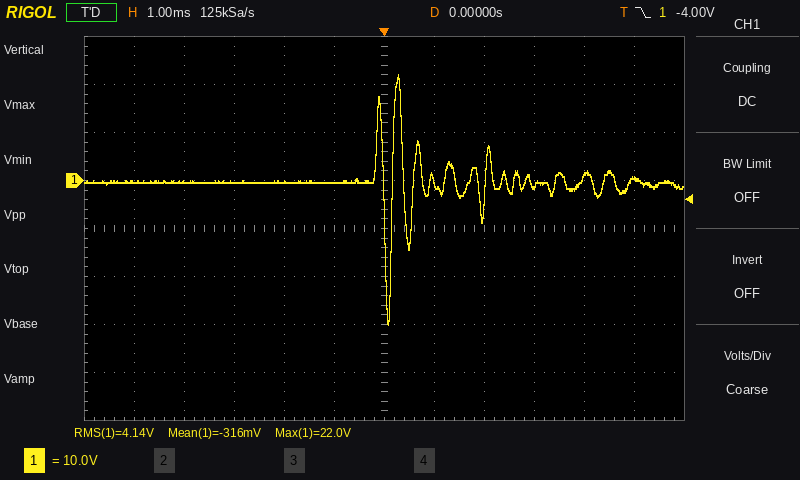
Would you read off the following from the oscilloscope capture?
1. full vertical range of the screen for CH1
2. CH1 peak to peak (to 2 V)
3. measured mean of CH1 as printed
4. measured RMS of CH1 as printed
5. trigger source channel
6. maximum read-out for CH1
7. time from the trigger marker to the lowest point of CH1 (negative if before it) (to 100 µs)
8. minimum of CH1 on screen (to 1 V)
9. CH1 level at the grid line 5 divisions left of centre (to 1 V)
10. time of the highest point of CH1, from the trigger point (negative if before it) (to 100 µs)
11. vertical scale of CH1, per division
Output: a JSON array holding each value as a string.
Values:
["80 V", "52 V", "-316 mV", "4.14 V", "CH1", "22.0 V", "+100 µs", "-30 V", "0 V", "+300 µs", "10 V"]
